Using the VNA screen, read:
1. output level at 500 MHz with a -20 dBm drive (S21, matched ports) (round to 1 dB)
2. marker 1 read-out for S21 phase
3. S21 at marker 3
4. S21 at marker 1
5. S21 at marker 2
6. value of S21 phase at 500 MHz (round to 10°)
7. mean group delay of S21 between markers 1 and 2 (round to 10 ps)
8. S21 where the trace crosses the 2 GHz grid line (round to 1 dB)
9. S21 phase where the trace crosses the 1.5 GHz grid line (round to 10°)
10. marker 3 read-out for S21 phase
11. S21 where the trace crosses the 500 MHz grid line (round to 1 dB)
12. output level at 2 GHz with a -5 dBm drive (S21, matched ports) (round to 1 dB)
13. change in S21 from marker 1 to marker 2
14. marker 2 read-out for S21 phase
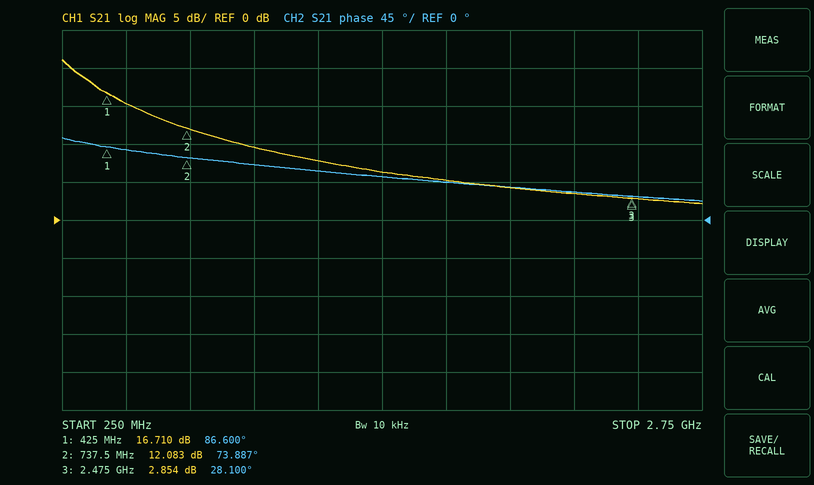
-5 dBm
86.600°
2.854 dB
16.710 dB
12.083 dB
80°
110 ps
4 dB
50°
28.100°
15 dB
-1 dBm
-4.627 dB
73.887°
